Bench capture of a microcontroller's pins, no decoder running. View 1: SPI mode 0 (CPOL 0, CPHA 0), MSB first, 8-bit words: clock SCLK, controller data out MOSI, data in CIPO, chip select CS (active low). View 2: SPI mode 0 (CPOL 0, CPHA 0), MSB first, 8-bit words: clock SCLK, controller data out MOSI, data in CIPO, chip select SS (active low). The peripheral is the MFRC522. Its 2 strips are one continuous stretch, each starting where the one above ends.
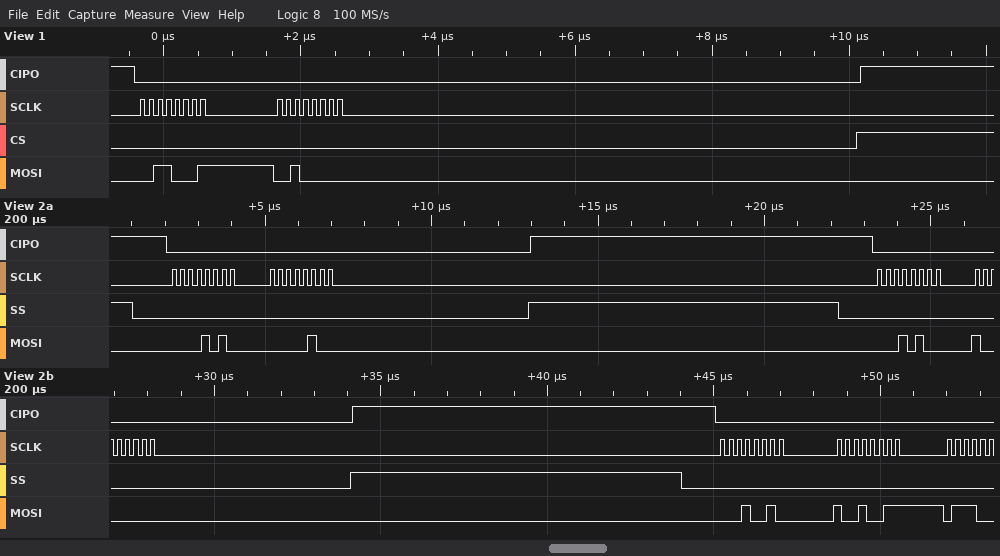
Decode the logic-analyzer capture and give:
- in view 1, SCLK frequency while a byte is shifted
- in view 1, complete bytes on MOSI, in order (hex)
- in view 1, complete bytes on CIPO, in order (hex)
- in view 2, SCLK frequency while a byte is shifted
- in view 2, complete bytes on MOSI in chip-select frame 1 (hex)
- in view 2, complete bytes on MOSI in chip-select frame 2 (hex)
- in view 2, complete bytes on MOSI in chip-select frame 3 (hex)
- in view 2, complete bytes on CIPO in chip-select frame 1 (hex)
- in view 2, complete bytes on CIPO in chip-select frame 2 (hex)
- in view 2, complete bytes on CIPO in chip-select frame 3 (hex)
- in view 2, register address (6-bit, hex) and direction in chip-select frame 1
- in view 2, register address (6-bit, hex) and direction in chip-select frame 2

8 MHz
31 20
00 00
4 MHz
0A 04
14 80
12 93
00 00
00 00
00 00
0x05 write
0x0A write
